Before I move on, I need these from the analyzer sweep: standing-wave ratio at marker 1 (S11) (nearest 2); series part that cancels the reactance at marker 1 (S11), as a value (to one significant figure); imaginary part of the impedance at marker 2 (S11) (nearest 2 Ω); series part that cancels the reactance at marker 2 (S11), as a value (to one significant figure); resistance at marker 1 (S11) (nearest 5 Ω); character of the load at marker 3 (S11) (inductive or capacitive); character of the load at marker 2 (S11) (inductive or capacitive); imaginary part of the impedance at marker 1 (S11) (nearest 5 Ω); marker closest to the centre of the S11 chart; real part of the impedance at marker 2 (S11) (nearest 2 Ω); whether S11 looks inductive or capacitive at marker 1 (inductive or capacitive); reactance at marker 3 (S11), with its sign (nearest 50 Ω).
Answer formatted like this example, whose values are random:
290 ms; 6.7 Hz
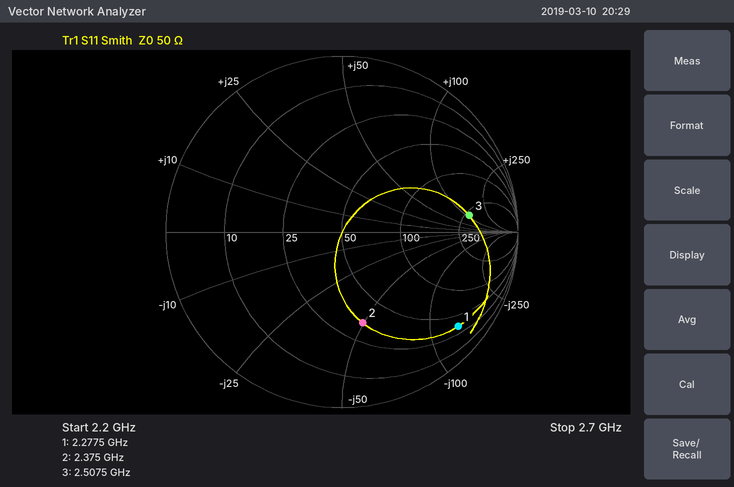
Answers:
12; 9 nH; -50 Ω; 3 nH; 35 Ω; inductive; capacitive; -135 Ω; marker 2; 34 Ω; capacitive; +100 Ω
